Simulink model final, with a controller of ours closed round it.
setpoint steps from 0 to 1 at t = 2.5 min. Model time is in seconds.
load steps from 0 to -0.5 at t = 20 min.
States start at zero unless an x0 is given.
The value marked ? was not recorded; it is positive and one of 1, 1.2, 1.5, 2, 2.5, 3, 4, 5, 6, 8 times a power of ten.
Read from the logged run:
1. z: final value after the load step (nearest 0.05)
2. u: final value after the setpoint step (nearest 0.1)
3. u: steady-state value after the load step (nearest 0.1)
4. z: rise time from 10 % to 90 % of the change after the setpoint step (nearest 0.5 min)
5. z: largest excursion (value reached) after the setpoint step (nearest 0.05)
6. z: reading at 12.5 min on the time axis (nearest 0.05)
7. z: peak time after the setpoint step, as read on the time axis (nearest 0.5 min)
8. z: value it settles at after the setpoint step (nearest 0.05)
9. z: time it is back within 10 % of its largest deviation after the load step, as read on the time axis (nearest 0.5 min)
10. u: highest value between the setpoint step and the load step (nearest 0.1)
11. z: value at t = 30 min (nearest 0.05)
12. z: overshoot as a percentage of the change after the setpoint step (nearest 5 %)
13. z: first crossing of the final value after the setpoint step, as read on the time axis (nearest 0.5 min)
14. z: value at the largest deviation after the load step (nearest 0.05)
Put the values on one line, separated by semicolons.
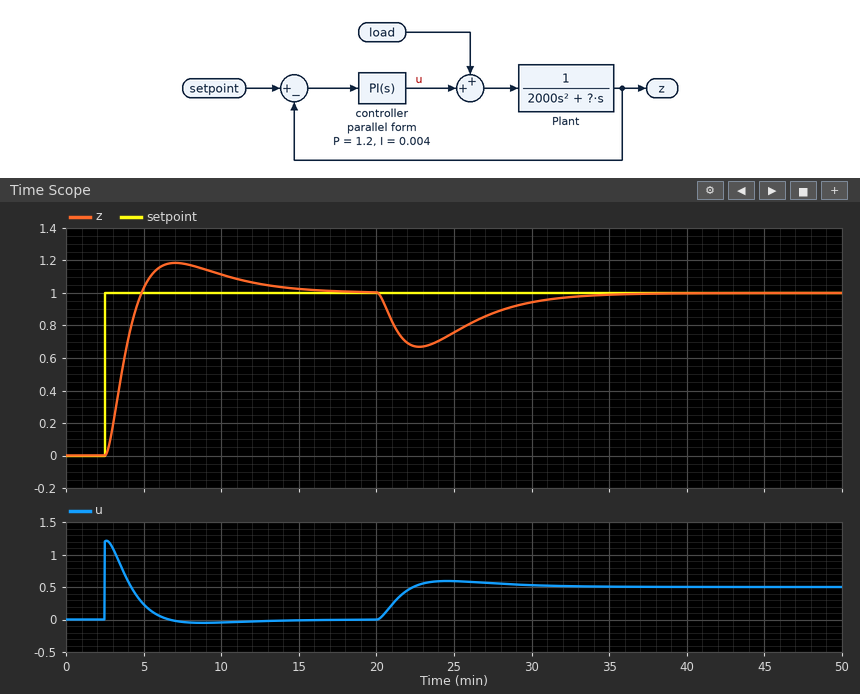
1.00; 0.0; 0.5; 1.5 min; 1.20; 1.05; 7.0 min; 1.00; 31.5 min; 1.2; 0.95; 20 %; 5.0 min; 0.65
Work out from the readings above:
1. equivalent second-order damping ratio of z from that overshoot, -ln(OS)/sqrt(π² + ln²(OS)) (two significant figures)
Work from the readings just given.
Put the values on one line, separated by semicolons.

0.46
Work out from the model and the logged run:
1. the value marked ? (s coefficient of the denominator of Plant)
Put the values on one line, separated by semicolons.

100
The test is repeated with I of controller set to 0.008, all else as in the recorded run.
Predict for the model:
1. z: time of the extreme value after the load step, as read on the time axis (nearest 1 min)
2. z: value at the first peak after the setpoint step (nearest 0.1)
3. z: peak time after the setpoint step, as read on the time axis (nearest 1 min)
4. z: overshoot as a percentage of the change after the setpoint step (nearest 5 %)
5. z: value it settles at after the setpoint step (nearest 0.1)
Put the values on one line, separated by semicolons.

22 min; 1.3; 6 min; 30 %; 1.0
